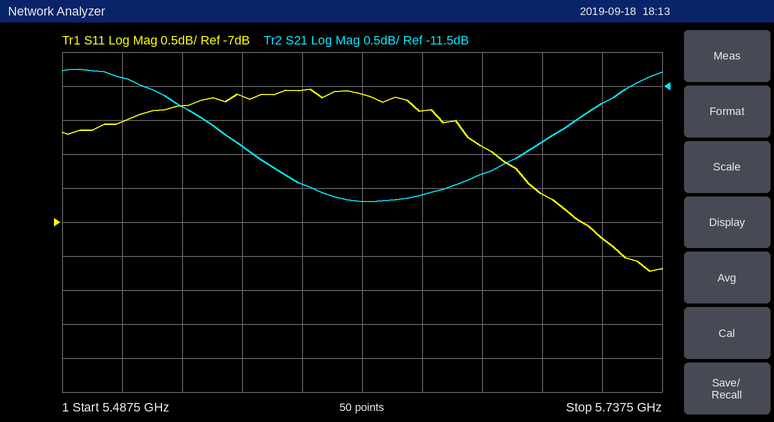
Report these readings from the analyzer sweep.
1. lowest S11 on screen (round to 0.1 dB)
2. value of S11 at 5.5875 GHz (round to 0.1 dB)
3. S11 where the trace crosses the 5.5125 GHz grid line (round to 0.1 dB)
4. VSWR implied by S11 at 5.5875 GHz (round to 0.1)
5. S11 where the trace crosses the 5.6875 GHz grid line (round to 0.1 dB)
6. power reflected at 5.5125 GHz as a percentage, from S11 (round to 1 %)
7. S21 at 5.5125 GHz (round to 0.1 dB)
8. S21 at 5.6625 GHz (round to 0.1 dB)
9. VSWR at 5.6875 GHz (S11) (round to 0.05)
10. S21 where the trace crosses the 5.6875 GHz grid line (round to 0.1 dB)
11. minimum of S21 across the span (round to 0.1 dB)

-7.7 dB
-5.1 dB
-5.5 dB
3.5
-6.6 dB
28 %
-11.4 dB
-12.8 dB
2.75
-12.3 dB
-13.2 dB
